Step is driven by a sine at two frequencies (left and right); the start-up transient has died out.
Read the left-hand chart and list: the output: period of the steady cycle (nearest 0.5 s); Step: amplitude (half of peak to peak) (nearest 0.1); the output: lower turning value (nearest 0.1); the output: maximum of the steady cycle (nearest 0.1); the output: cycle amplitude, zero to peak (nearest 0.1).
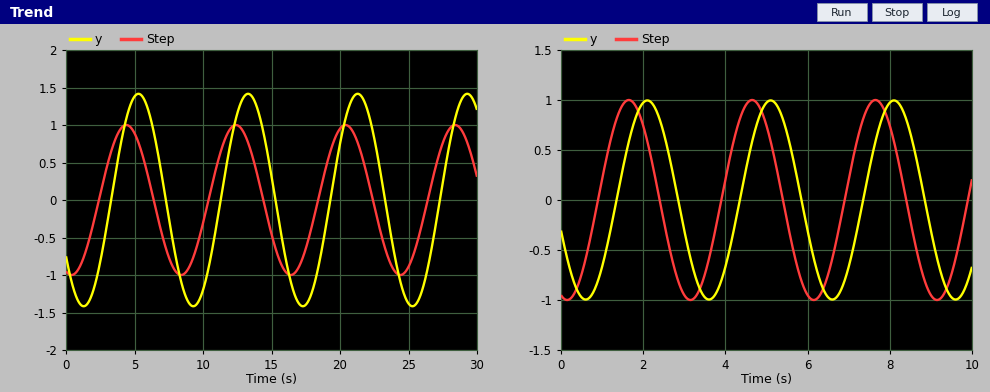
8.0 s
1.0
-1.4
1.4
1.4
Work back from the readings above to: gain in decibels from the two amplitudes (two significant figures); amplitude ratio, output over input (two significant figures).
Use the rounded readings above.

2.9 dB
1.4
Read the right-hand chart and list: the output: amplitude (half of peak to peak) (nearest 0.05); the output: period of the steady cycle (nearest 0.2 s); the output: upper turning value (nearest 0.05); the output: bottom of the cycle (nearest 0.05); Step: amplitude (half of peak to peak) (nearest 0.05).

1.00
3.0 s
1.00
-1.00
1.00
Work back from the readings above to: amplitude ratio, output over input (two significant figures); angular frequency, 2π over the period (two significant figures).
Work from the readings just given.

1.0
2.1 rad/s
